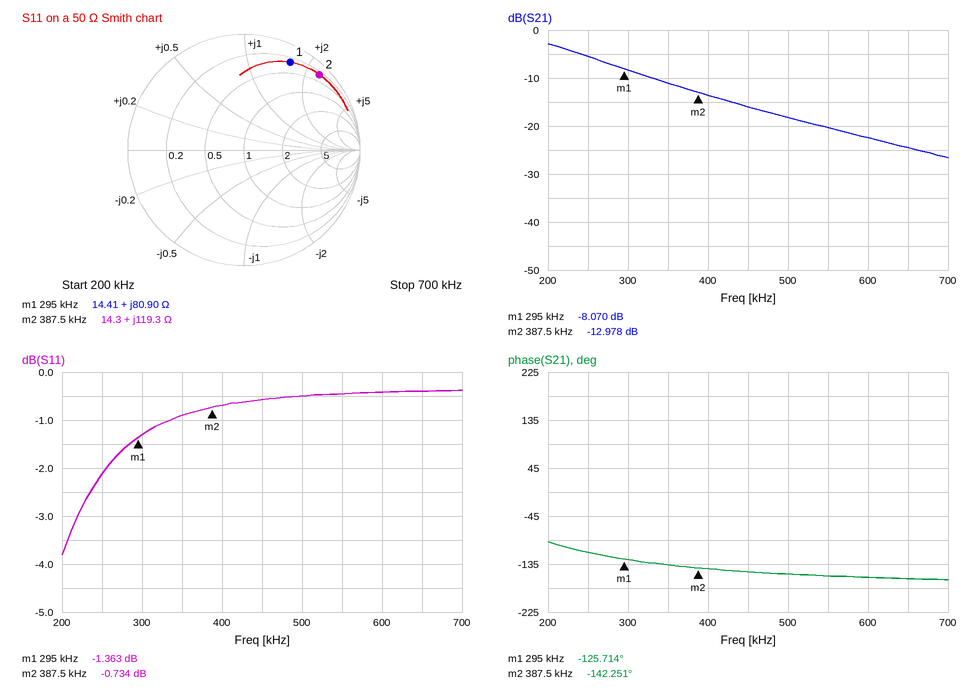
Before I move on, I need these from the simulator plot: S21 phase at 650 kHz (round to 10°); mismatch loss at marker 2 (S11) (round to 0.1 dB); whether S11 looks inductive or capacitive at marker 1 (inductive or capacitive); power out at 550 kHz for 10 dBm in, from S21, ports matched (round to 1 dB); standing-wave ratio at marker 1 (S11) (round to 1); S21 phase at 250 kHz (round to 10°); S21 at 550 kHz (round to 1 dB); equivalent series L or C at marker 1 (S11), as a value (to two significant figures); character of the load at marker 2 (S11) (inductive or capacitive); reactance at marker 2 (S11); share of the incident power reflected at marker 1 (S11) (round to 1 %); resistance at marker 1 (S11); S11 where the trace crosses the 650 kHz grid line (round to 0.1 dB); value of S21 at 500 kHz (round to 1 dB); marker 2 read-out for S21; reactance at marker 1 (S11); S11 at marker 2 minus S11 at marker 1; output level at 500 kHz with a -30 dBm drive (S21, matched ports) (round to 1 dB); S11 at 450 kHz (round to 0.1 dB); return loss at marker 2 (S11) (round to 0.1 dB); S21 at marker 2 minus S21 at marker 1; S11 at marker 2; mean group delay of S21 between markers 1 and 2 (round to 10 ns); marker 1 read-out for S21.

-160°
8.1 dB
inductive
-10 dBm
13
-110°
-20 dB
44 µH
inductive
+119.3 Ω
73 %
14.41 Ω
-0.4 dB
-18 dB
-12.978 dB
+80.90 Ω
0.629 dB
-48 dBm
-0.6 dB
0.7 dB
-4.908 dB
-0.734 dB
500 ns
-8.070 dB
